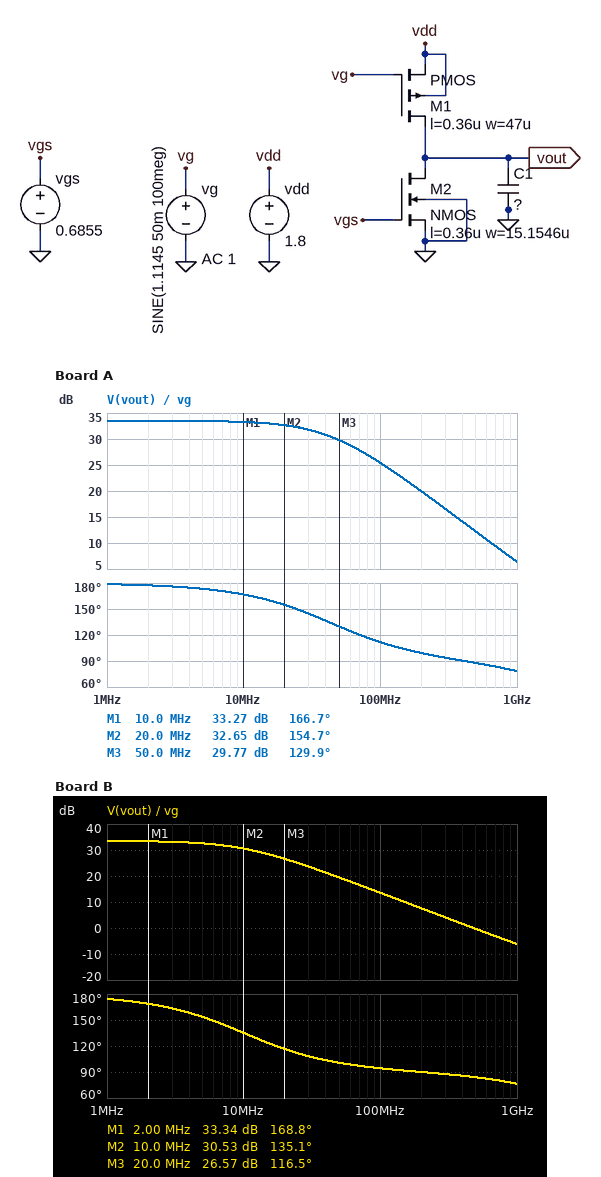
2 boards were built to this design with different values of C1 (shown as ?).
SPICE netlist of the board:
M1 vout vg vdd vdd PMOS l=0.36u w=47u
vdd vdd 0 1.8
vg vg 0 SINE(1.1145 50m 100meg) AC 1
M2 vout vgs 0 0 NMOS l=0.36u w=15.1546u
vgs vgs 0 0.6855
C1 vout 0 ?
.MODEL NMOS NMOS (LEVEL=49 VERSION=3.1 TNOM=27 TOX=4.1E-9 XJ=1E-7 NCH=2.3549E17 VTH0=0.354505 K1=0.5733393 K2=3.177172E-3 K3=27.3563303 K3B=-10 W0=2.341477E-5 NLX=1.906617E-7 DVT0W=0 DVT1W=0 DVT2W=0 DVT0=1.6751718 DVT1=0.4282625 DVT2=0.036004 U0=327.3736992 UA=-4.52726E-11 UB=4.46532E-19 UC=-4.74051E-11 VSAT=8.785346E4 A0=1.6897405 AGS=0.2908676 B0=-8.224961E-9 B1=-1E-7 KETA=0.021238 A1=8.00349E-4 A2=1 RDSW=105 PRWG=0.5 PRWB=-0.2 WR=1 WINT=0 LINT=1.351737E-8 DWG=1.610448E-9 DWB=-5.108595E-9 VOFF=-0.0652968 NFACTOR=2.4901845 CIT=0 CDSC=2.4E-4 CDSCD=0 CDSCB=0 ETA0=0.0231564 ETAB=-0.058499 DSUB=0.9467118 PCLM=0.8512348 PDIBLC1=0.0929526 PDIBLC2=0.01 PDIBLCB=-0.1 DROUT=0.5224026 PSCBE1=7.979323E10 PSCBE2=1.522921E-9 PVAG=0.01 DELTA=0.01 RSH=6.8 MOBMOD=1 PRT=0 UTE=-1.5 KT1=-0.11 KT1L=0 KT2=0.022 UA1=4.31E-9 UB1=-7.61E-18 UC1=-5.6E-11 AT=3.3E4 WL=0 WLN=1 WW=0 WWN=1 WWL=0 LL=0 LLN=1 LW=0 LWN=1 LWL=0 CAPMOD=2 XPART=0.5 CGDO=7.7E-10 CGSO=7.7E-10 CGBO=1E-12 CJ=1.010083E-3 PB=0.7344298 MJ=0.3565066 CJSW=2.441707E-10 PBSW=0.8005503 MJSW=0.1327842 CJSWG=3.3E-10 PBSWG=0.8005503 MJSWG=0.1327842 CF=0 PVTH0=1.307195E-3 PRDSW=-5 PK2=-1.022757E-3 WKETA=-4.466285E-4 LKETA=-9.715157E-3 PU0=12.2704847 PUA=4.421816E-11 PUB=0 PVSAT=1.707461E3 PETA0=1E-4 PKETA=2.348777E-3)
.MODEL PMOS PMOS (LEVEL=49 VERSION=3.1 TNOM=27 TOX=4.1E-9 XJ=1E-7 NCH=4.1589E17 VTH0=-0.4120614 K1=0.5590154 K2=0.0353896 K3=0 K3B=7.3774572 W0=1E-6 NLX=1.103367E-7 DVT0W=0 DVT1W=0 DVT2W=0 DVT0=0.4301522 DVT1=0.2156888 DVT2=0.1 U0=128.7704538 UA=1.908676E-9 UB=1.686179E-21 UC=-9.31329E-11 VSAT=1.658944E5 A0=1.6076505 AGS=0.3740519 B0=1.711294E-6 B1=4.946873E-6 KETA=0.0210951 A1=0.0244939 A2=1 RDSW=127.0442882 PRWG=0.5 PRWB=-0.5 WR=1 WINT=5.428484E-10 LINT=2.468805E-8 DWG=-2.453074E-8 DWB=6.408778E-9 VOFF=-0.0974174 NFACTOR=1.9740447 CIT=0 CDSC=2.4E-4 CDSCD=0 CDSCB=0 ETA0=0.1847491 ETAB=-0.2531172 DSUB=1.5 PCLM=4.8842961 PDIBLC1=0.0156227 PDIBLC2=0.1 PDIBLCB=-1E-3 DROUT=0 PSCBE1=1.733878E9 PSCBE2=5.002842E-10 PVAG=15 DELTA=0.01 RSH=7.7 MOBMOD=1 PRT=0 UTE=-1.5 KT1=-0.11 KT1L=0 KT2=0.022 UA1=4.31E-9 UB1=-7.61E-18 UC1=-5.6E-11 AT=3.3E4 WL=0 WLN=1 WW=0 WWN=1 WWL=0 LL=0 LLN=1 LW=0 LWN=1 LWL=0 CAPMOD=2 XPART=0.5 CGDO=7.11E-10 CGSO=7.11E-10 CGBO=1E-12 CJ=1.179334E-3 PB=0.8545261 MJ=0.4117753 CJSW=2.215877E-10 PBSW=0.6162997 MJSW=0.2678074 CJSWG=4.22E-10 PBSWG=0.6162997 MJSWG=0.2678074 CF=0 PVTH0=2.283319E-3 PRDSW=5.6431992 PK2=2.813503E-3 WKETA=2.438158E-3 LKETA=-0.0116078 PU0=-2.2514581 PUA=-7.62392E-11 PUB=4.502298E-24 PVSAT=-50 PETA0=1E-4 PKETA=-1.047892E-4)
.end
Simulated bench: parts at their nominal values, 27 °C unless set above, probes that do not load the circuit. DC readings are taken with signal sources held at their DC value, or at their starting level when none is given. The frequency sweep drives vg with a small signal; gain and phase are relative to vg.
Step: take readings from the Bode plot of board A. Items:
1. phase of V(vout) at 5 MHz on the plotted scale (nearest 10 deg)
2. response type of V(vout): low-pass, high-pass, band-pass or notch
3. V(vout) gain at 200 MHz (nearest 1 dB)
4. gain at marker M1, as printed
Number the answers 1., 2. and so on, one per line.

1. 170 deg
2. low-pass
3. 20 dB
4. 33.27 dB
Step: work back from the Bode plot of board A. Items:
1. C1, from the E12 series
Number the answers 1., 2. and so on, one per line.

1. 82 fF
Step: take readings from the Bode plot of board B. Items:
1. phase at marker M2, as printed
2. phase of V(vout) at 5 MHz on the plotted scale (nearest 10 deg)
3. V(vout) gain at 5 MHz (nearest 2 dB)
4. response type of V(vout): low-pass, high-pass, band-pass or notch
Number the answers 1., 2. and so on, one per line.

1. 135.1 deg
2. 150 deg
3. 32 dB
4. low-pass
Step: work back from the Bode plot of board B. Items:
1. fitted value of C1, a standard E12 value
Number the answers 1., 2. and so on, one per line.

1. 560 fF
